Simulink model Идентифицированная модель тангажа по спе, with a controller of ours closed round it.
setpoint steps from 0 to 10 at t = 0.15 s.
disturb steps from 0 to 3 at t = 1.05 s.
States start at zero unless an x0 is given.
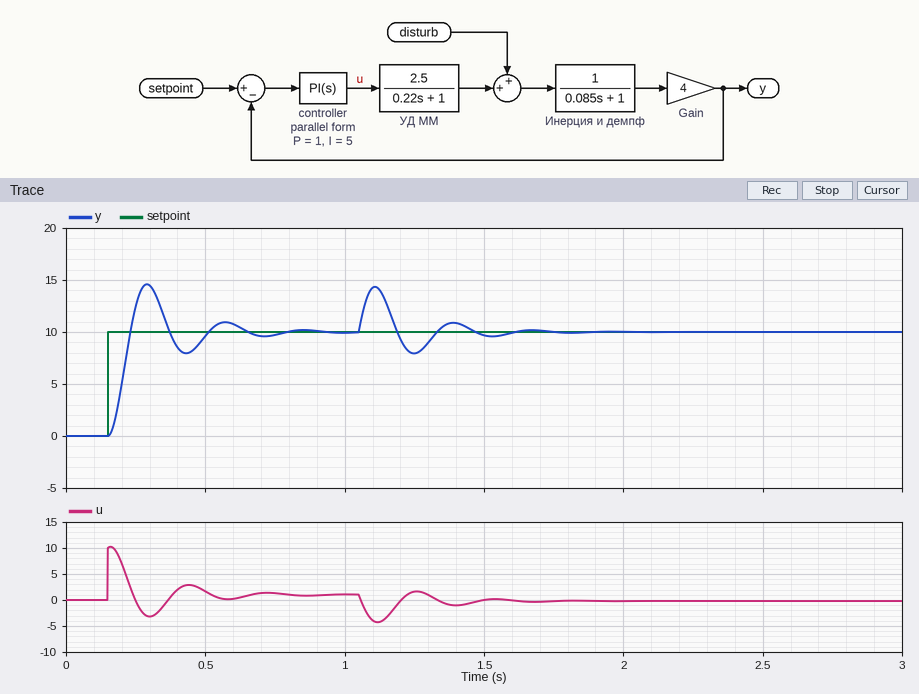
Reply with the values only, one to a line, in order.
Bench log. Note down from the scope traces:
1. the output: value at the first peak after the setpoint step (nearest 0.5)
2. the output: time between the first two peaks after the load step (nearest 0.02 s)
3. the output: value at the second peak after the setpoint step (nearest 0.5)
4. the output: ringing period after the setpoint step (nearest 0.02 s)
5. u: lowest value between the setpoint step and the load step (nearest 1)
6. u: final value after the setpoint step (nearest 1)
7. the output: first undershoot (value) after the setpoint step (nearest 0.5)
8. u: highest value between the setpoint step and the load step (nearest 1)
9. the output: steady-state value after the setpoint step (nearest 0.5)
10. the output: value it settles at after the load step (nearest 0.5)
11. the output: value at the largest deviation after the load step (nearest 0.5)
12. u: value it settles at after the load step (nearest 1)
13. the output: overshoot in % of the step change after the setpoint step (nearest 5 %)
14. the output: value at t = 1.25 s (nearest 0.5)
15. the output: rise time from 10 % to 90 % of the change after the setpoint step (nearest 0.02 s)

14.5
0.28 s
11.0
0.28 s
-3
1
8.0
10
10.0
10.0
14.5
0
45 %
8.0
0.06 s
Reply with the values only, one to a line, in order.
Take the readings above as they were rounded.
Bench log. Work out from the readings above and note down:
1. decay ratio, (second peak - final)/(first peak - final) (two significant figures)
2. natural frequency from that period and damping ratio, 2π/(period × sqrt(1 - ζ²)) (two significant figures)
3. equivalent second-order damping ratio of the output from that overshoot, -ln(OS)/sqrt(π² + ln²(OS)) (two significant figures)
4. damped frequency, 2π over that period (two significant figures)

0.22
23 rad/s
0.25
22 rad/s
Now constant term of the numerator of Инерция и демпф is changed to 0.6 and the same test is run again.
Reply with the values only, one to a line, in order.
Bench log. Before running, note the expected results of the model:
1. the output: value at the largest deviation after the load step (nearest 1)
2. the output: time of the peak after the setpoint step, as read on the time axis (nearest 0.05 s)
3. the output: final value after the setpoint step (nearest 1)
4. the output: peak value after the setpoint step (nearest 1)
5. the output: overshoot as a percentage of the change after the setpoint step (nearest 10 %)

13
0.35 s
10
14
40 %
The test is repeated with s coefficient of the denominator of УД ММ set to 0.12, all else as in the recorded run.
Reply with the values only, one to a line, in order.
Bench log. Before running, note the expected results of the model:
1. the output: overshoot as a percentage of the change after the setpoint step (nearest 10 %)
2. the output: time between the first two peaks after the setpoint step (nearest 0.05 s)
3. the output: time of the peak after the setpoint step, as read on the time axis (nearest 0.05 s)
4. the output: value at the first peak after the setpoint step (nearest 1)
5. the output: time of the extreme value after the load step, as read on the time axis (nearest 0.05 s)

40 %
0.20 s
0.25 s
14
1.10 s
